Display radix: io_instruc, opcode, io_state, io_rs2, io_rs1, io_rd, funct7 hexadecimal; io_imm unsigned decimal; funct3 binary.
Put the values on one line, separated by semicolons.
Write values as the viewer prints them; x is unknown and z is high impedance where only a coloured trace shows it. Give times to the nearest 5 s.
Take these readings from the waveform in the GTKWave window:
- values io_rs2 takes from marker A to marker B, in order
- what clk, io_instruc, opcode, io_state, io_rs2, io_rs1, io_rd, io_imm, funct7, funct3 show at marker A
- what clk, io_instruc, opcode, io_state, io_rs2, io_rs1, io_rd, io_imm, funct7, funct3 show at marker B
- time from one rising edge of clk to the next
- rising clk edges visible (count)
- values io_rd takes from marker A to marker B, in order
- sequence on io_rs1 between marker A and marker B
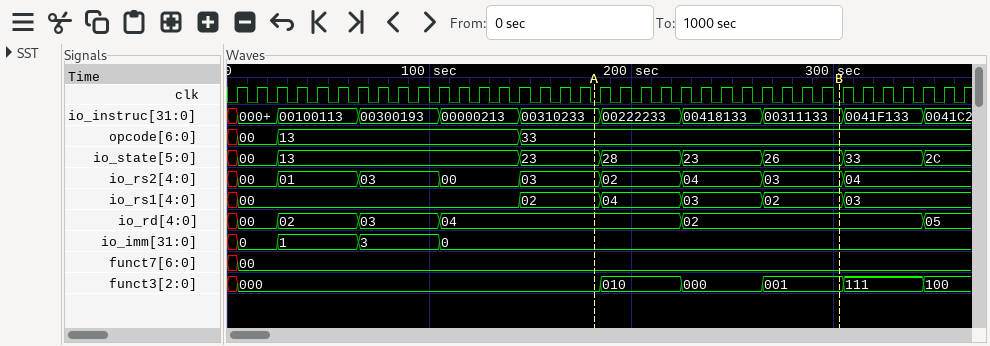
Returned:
03, 02, 04, 03; clk=0, io_instruc=00310233, opcode=33, io_state=23, io_rs2=03, io_rs1=02, io_rd=04, io_imm=0, funct7=00, funct3=000; clk=0, io_instruc=00311133, opcode=33, io_state=26, io_rs2=03, io_rs1=02, io_rd=02, io_imm=0, funct7=00, funct3=001; 10 s; 37; 04, 02; 02, 04, 03, 02
